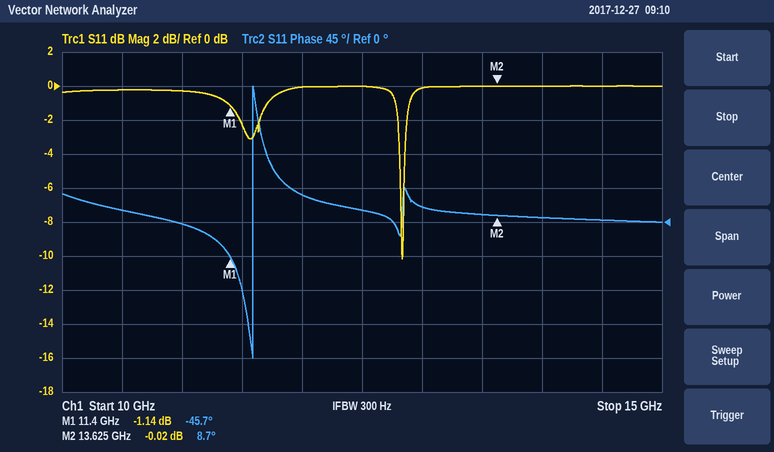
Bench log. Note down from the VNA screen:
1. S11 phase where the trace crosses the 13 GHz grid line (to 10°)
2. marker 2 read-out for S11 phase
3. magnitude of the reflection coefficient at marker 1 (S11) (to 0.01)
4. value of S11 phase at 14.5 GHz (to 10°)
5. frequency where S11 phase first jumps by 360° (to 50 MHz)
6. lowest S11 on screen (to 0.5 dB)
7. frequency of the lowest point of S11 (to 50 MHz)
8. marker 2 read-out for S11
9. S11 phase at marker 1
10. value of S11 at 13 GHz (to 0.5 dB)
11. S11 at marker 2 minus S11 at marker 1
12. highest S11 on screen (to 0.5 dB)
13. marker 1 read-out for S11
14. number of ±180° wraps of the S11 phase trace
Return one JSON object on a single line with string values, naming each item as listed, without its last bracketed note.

{"S11 phase where the trace crosses the 13 GHz grid line": "20°", "marker 2 read-out for S11 phase": "8.7°", "magnitude of the reflection coefficient at marker 1 (S11)": "0.88", "value of S11 phase at 14.5 GHz": "0°", "frequency where S11 phase first jumps by 360°": "11.60 GHz", "lowest S11 on screen": "-10.0 dB", "frequency of the lowest point of S11": "12.85 GHz", "marker 2 read-out for S11": "-0.02 dB", "S11 phase at marker 1": "-45.7°", "value of S11 at 13 GHz": "0.0 dB", "S11 at marker 2 minus S11 at marker 1": "1.12 dB", "highest S11 on screen": "0.0 dB", "marker 1 read-out for S11": "-1.14 dB", "number of ±180° wraps of the S11 phase trace": "1"}
